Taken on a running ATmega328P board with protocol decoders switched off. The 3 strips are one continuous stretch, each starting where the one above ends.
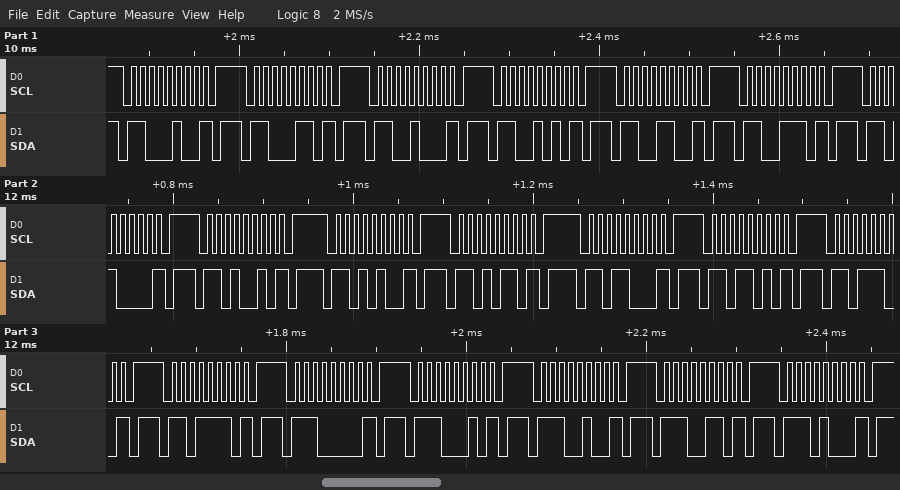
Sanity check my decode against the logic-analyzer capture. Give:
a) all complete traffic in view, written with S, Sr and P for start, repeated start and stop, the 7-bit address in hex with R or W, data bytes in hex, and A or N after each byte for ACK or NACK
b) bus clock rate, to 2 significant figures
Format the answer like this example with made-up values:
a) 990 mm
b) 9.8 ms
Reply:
a) S 62W N P S 63W N P S 64W N P S 65W N P S 66W N P S 67W N P S 68W N P S 69W N P S 6AW N P S 6BW N P S 6CW N P S 6DW N P S 6EW N P S 6FW N P S 70W N P S 71W N P S 72W N P S 73W N P S 74W N P
b) 100 kHz
